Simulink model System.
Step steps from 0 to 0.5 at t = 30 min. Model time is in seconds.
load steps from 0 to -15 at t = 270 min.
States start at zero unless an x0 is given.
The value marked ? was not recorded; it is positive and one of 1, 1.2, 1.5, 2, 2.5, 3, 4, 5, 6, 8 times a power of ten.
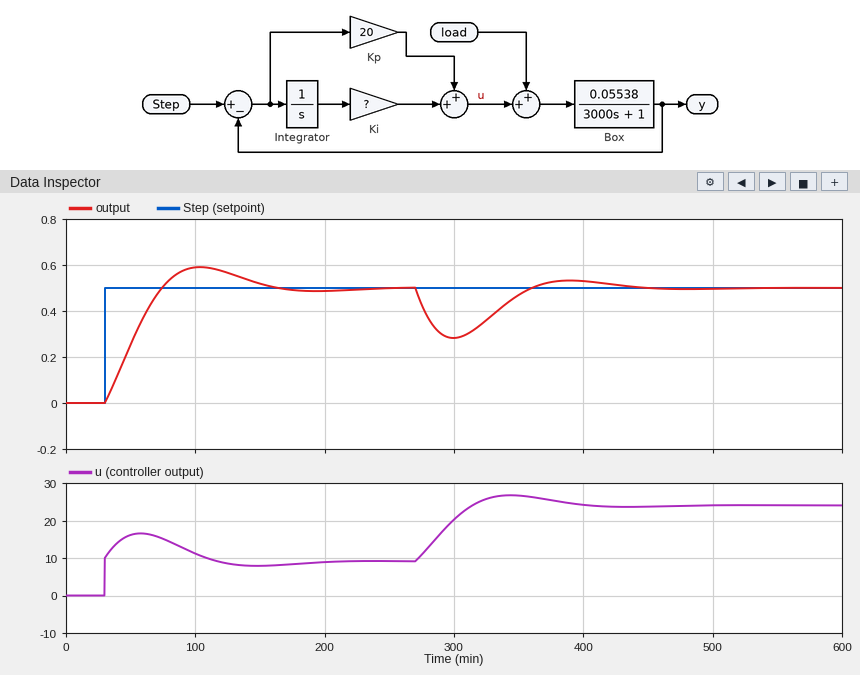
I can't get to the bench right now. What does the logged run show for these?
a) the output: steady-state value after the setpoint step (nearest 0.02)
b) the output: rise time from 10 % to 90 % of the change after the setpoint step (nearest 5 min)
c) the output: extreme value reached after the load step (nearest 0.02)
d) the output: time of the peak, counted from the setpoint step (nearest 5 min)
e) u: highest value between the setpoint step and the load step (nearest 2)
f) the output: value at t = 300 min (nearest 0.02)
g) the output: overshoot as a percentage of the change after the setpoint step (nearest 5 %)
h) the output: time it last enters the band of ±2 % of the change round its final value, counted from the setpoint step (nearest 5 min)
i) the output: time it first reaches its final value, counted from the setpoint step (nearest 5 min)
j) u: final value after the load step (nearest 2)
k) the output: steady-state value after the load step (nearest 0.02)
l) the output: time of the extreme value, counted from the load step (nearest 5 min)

0.50
35 min
0.28
75 min
16
0.28
20 %
185 min
45 min
24
0.50
30 min
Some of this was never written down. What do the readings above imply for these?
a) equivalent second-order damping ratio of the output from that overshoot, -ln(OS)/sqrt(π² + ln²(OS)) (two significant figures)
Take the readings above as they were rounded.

0.46
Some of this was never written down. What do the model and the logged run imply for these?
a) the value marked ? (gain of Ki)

0.025
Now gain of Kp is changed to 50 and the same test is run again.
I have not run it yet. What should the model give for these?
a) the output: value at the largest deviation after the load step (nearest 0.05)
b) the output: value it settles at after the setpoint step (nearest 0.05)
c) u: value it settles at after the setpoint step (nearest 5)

0.35
0.50
10
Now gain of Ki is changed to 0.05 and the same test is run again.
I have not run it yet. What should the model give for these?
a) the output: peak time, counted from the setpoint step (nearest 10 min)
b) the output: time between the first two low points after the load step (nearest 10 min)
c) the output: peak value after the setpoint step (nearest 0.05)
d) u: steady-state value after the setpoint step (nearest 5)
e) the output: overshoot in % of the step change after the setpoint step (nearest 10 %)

50 min
120 min
0.65
10
30 %
